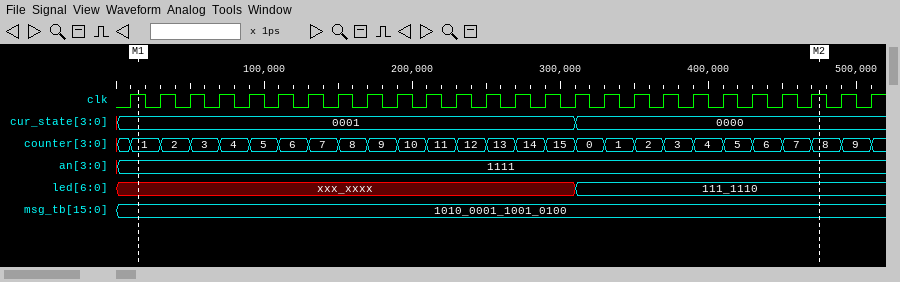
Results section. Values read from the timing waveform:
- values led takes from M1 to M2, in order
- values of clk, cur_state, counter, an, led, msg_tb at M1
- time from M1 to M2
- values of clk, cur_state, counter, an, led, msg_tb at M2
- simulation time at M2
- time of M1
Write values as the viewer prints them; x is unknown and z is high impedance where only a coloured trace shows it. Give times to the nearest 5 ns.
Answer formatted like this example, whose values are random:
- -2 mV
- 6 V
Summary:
- xxx_xxxx, 111_1110
- clk=1, cur_state=0001, counter=1, an=1111, led=xxx_xxxx, msg_tb=1010_0001_1001_0100
- 460 ns
- clk=1, cur_state=0000, counter=8, an=1111, led=111_1110, msg_tb=1010_0001_1001_0100
- 475 ns
- 15 ns
